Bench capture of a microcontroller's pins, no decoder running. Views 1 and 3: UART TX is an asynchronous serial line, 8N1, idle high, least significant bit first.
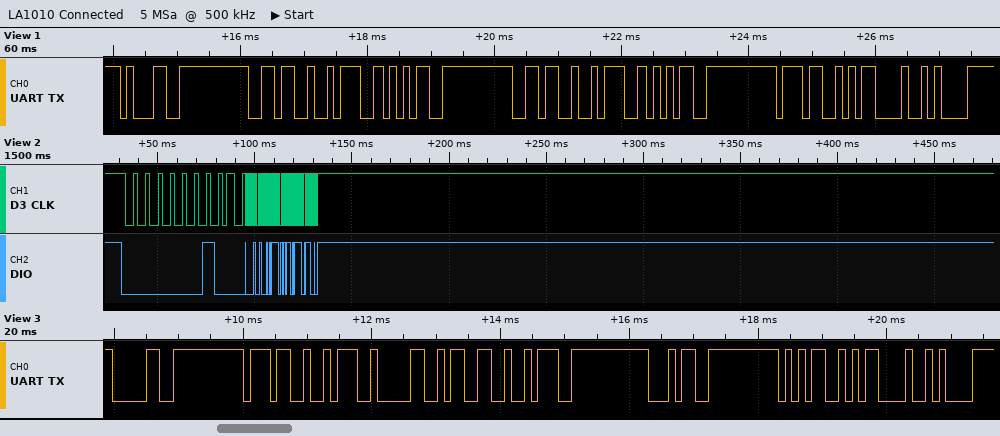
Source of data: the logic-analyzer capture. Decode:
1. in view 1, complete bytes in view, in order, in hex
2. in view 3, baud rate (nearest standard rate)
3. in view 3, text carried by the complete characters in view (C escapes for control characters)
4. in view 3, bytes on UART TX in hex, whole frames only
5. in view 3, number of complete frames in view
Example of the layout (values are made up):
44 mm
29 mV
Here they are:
31 36 3A 35 36 3A 35 37 0D 0A
9600 baud
"07:03:45\r\n"
30 37 3A 30 33 3A 34 35 0D 0A
10
